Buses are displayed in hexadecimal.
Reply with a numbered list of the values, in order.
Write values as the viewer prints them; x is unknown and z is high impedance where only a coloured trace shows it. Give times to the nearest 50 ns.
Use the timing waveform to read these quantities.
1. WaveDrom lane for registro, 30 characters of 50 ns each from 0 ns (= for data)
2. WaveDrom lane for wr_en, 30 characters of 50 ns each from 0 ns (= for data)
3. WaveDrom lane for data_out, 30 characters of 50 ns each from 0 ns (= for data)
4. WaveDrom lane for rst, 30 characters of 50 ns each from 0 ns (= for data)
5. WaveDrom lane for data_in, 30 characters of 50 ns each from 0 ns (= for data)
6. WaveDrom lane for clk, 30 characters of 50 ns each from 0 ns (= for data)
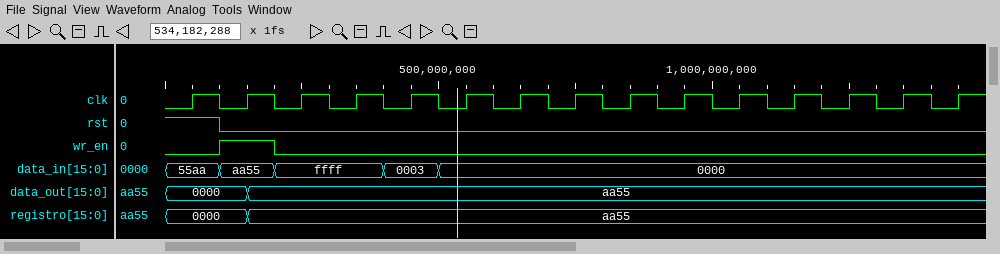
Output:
1. {name: 'registro', wave: '=..=..........................', data: '0000 aa55'}
2. {name: 'wr_en', wave: '0.1.0.........................'}
3. {name: 'data_out', wave: '=..=..........................', data: '0000 aa55'}
4. {name: 'rst', wave: '1.0...........................'}
5. {name: 'data_in', wave: '=.=.=...=.=...................', data: '55aa aa55 ffff 0003 0000'}
6. {name: 'clk', wave: '010101010101010101010101010101'}
